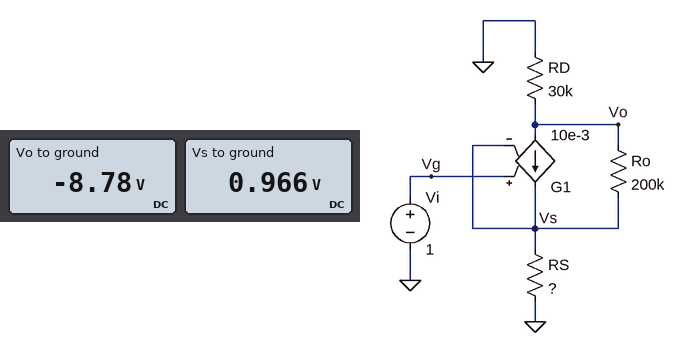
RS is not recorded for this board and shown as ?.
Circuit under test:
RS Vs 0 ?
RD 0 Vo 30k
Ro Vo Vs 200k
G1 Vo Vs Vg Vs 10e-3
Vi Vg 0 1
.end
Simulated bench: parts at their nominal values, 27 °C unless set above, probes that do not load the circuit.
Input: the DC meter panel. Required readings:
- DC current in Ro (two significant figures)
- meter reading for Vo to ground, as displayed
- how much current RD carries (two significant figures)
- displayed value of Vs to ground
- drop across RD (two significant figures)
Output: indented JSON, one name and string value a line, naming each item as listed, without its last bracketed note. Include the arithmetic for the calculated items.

{
  "DC current in Ro": "(966 mV - (-8.78 V)) / 200 kΩ = 49 µA",
  "meter reading for Vo to ground, as displayed": "-8.78 V",
  "how much current RD carries": "(0 V - (-8.78 V)) / 30 kΩ = 290 µA",
  "displayed value of Vs to ground": "0.966 V",
  "drop across RD": "0 V - (-8.78 V) = 8.8 V"
}
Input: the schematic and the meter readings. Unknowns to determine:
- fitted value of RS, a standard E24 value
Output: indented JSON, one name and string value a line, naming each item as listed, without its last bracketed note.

{
  "fitted value of RS, a standard E24 value": "3.3 kΩ"
}
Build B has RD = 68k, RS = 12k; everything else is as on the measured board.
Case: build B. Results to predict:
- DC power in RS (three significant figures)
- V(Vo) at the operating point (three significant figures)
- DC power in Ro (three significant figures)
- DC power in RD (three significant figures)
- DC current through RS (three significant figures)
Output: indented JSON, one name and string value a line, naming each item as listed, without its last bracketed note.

{
  "DC power in RS": "81.4 µW",
  "V(Vo) at the operating point": "-5.60 V",
  "DC power in Ro": "217 µW",
  "DC power in RD": "461 µW",
  "DC current through RS": "82.4 µA"
}
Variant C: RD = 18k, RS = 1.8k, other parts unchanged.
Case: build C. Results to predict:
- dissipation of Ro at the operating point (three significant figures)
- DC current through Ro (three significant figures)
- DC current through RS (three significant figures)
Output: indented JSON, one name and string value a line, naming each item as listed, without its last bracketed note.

{
  "dissipation of Ro at the operating point": "537 µW",
  "DC current through Ro": "51.8 µA",
  "DC current through RS": "524 µA"
}
